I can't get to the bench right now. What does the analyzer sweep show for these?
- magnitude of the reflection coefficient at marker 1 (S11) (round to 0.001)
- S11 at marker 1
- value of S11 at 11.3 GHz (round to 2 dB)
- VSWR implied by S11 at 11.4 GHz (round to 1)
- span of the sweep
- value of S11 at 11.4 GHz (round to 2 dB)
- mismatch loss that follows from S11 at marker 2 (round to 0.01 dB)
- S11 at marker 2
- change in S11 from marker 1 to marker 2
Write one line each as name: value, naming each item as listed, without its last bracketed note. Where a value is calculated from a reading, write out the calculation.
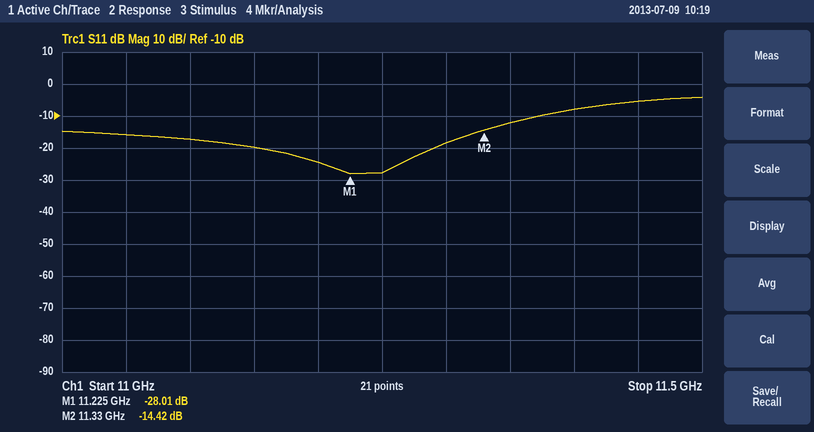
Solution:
magnitude of the reflection coefficient at marker 1 (S11): 10^(-28.01/20) ≈ 0.040
S11 at marker 1: -28.01 dB
value of S11 at 11.3 GHz: -18 dB
VSWR implied by S11 at 11.4 GHz: |Γ| = 10^(-8/20) = 0.3981; VSWR = (1 + 0.3981)/(1 − 0.3981) ≈ 2
span of the sweep: 500 MHz
value of S11 at 11.4 GHz: -8 dB
mismatch loss that follows from S11 at marker 2: −10 log10(1 − 10^(-14.42/10)) ≈ 0.16 dB
S11 at marker 2: -14.42 dB
change in S11 from marker 1 to marker 2: -14.42 − (-28.01) = 13.59 dB
